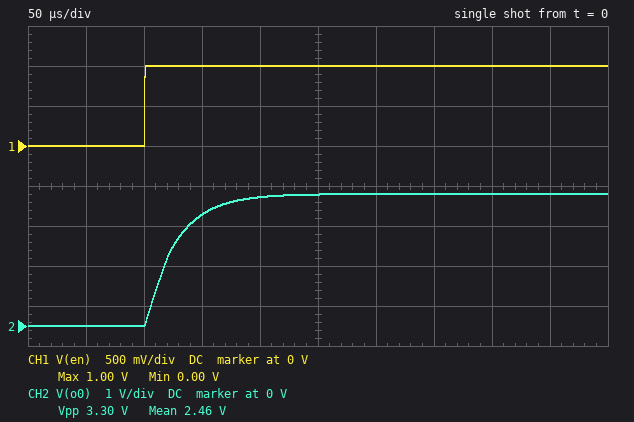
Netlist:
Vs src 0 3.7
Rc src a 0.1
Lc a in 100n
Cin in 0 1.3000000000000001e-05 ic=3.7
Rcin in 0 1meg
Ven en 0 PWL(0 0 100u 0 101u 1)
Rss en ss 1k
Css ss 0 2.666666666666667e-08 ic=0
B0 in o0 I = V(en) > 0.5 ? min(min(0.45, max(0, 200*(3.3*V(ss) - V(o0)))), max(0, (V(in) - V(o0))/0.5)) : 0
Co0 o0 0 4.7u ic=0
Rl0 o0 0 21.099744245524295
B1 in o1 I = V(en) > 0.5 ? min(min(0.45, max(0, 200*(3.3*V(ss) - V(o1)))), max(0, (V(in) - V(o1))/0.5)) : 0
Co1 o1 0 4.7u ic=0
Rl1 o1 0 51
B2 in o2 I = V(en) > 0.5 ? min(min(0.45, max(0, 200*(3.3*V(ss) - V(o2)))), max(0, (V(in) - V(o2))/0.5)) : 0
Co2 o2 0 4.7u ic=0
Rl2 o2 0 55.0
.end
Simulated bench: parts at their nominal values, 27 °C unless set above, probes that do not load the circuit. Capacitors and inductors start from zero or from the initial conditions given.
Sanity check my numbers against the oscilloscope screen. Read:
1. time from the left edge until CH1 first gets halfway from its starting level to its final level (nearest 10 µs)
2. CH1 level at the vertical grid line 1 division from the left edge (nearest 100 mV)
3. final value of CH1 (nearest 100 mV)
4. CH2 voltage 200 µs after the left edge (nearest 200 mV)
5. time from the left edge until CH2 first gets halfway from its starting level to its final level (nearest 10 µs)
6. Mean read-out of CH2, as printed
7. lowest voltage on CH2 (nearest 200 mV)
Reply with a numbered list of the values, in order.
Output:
1. 100 µs
2. 0 V
3. 1.0 V
4. 3.2 V
5. 120 µs
6. 2.46 V
7. 0 V
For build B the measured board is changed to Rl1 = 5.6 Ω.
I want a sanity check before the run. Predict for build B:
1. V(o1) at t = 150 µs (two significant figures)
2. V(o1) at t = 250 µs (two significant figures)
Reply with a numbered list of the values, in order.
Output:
1. 2.1 V
2. 2.5 V
